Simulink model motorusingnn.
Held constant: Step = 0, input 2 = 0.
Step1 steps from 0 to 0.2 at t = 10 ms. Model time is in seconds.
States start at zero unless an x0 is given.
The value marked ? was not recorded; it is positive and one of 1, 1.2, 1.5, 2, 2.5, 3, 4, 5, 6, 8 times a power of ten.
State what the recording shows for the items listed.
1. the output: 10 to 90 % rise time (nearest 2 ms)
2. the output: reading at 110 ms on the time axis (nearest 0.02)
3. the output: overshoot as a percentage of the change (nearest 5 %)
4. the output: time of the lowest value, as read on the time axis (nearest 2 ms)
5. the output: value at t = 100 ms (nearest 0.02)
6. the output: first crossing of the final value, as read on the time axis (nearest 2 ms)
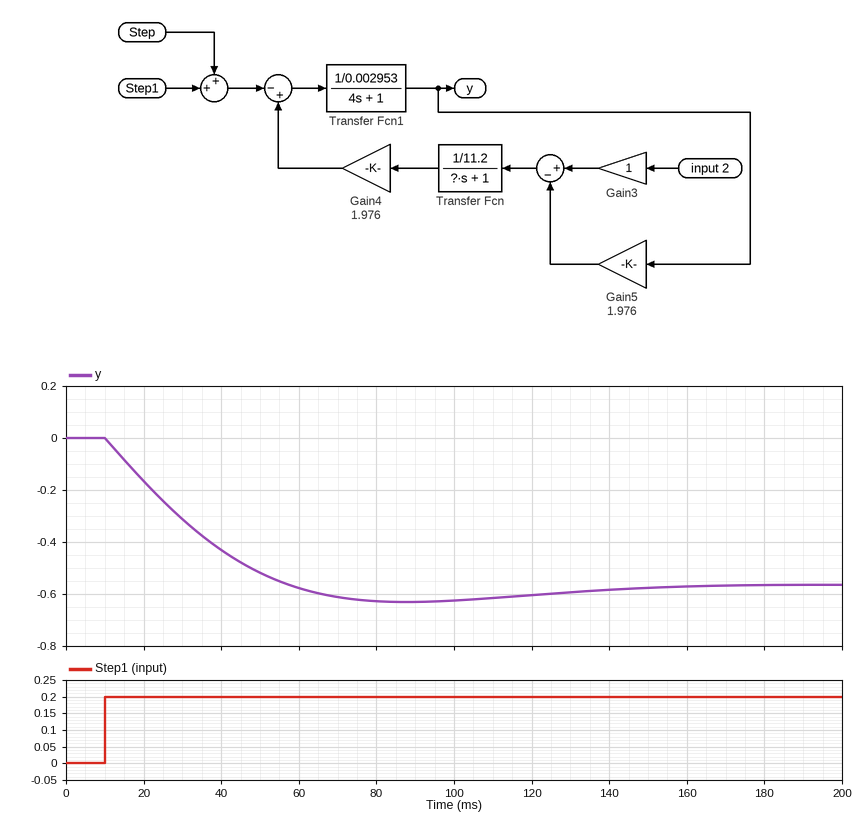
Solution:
36 ms
-0.62
10 %
88 ms
-0.62
58 ms
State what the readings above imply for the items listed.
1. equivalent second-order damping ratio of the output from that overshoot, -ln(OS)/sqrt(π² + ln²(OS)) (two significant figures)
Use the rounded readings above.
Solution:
0.59
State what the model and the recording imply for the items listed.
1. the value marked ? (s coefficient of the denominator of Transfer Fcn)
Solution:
0.02
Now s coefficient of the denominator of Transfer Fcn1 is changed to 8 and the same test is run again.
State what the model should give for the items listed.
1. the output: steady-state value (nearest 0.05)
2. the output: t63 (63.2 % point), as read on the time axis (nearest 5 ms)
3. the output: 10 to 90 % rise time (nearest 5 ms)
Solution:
-0.55
60 ms
95 ms
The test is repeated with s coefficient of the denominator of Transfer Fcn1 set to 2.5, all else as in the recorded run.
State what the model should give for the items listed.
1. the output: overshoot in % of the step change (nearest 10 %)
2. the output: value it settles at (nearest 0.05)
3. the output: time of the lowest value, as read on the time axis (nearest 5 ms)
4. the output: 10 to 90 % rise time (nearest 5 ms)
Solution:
30 %
-0.55
60 ms
20 ms
